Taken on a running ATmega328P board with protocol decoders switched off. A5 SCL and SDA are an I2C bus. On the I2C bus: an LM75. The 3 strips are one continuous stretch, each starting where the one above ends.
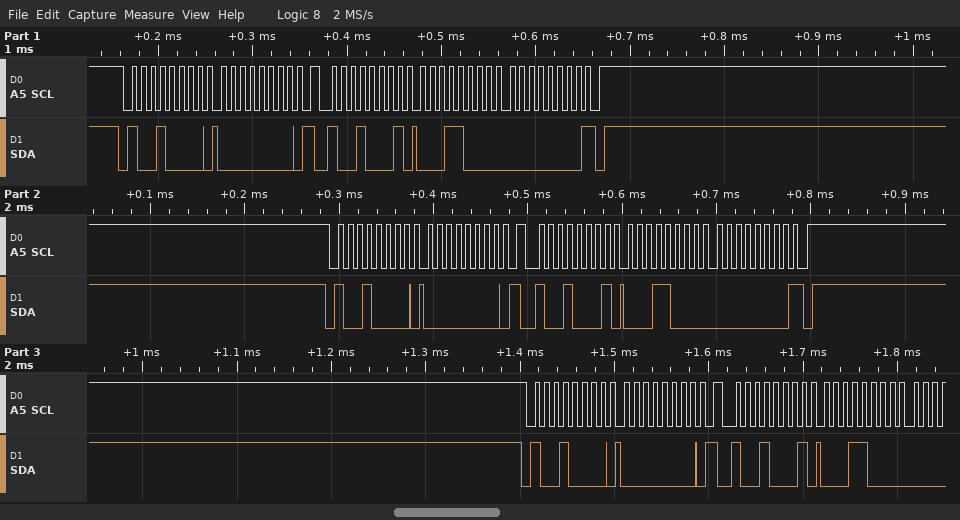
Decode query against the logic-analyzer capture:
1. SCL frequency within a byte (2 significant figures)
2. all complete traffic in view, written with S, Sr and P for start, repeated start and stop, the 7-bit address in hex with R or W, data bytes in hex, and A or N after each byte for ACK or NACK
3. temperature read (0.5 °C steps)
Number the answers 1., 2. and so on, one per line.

1. 100 kHz
2. S 48W A 00 A Sr 48R A 18 A 00 N P S 48W A 00 A Sr 48R A 18 A 00 N P S 48W A 00 A Sr 48R A 18 A
3. 24.0 °C
